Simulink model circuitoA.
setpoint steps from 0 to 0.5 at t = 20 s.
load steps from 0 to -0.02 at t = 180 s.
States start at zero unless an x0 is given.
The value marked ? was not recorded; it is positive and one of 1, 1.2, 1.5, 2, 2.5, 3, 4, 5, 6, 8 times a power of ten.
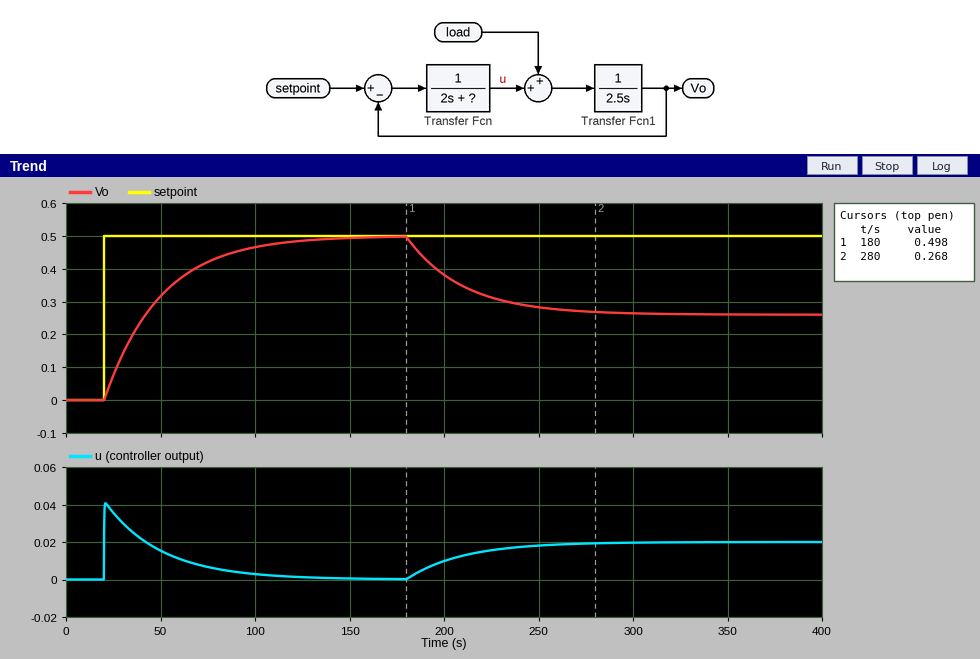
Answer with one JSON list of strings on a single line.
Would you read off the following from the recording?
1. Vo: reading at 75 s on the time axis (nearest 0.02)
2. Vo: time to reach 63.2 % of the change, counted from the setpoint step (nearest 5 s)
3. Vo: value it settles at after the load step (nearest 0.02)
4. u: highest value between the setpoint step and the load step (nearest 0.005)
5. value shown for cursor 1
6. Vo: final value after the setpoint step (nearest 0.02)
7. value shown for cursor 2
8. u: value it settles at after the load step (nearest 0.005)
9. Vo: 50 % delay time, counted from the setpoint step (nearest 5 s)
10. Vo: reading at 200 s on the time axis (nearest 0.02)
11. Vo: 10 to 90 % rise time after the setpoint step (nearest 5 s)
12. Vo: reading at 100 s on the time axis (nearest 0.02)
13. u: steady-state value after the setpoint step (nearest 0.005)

["0.42", "30 s", "0.26", "0.040", "0.498", "0.50", "0.268", "0.020", "20 s", "0.38", "65 s", "0.46", "0.000"]
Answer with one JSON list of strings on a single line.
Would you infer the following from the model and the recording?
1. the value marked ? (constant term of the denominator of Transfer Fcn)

["12"]
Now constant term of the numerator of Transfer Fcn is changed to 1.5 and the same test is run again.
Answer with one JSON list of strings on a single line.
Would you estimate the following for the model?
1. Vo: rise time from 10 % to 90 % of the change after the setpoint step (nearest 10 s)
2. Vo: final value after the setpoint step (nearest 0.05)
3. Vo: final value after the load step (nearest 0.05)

["40 s", "0.50", "0.35"]
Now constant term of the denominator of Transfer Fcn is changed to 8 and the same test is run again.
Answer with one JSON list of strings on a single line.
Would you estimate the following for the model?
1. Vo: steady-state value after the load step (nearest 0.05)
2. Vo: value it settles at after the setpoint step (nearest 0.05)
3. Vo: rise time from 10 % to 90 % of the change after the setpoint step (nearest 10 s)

["0.35", "0.50", "40 s"]
